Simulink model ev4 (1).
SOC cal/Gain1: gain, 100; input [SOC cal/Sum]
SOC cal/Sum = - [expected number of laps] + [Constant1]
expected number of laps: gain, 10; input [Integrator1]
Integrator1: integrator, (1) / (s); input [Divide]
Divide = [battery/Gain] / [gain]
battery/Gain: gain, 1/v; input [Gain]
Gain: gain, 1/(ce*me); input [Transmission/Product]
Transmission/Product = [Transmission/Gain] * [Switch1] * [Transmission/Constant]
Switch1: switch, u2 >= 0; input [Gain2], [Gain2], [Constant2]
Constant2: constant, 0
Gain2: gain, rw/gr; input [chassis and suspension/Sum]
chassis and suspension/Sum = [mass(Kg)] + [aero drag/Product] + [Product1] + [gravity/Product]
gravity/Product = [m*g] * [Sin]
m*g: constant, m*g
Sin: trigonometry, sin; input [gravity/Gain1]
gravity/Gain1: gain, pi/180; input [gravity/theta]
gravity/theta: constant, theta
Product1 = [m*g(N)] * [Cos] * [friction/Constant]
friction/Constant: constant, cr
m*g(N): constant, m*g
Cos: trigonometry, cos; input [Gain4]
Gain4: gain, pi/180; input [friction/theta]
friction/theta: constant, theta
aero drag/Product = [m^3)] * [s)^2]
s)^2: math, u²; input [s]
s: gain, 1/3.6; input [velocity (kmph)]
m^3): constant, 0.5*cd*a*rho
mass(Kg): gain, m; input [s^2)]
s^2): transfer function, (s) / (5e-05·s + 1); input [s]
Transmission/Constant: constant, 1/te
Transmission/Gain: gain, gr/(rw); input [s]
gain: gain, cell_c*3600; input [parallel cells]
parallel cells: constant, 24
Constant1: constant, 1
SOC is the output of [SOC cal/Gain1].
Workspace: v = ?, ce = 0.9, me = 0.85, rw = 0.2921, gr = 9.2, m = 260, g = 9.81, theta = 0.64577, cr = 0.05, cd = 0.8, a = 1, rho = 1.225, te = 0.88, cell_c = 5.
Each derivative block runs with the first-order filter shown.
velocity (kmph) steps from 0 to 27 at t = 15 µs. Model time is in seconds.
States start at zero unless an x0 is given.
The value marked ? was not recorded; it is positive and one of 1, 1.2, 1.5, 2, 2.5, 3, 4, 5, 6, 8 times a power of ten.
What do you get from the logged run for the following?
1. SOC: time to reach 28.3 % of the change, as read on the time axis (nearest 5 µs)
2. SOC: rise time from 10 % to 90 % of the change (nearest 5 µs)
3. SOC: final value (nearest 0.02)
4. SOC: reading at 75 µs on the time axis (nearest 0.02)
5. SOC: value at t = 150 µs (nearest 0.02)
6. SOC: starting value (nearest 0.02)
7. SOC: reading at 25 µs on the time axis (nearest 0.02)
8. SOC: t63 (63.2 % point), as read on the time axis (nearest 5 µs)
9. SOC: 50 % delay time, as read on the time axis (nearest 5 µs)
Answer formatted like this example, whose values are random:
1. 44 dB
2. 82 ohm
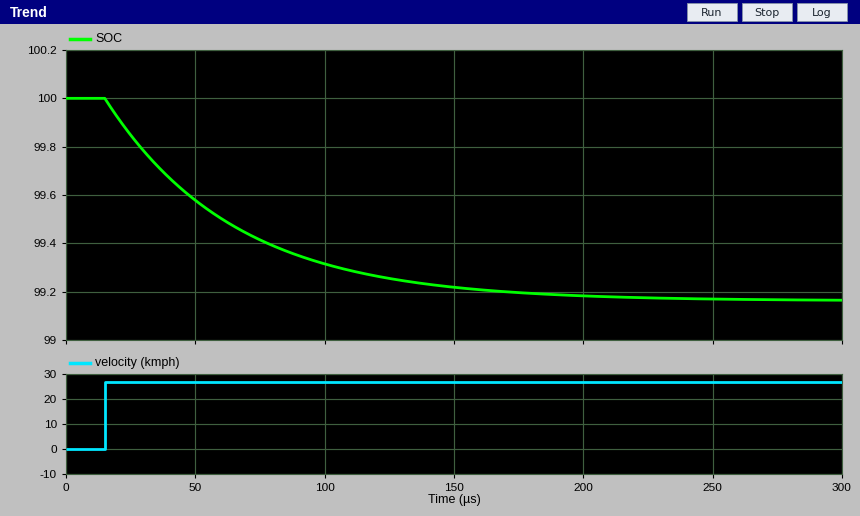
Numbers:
1. 30 µs
2. 110 µs
3. 99.16
4. 99.42
5. 99.22
6. 100.00
7. 99.84
8. 65 µs
9. 50 µs
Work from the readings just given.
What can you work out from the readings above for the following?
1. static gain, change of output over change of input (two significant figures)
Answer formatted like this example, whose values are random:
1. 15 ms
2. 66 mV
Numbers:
1. -0.031
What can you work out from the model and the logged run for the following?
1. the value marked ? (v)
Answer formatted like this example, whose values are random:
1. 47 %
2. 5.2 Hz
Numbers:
1. 60
